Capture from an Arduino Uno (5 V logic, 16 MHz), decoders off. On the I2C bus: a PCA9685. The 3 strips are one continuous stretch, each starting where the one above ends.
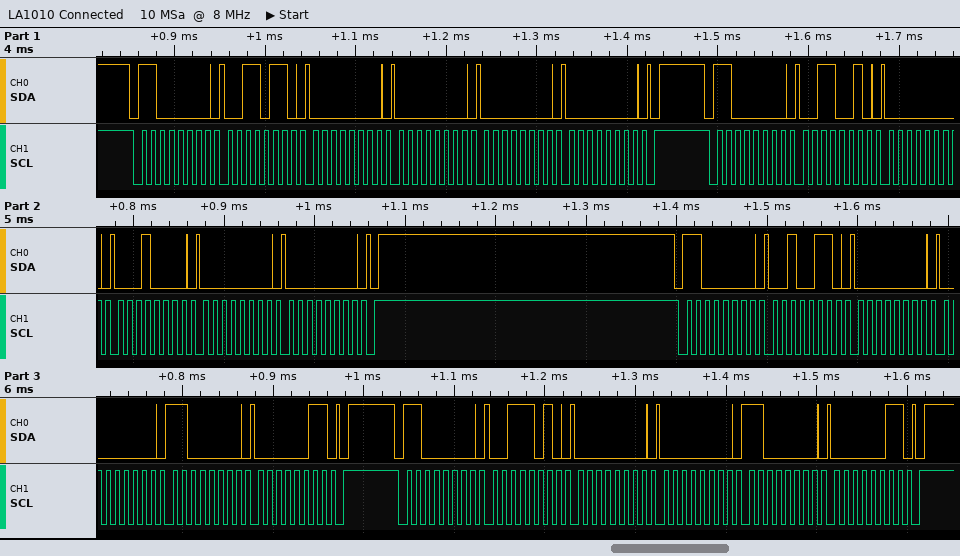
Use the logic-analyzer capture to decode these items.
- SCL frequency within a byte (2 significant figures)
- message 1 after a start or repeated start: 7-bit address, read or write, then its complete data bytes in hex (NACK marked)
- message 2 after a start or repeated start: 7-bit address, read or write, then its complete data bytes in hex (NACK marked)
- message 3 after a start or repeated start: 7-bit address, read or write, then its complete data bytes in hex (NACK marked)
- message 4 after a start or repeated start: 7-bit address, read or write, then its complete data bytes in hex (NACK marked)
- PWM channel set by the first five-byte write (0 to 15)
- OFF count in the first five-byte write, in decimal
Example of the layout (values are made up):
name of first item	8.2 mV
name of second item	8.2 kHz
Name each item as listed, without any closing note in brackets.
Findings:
SCL frequency within a byte	100 kHz
message 1 after a start or repeated start: 7-bit address, read or write, then its complete data bytes in hex	0x60 write: 36 00 00 00 00
message 2 after a start or repeated start: 7-bit address, read or write, then its complete data bytes in hex	0x60 write: 32 00 10 00 00
message 3 after a start or repeated start: 7-bit address, read or write, then its complete data bytes in hex	0x60 write: 26 00 00 C0 03
message 4 after a start or repeated start: 7-bit address, read or write, then its complete data bytes in hex	0x60 write: 3A 00 00 C0 03
PWM channel set by the first five-byte write	12
OFF count in the first five-byte write, in decimal	0
